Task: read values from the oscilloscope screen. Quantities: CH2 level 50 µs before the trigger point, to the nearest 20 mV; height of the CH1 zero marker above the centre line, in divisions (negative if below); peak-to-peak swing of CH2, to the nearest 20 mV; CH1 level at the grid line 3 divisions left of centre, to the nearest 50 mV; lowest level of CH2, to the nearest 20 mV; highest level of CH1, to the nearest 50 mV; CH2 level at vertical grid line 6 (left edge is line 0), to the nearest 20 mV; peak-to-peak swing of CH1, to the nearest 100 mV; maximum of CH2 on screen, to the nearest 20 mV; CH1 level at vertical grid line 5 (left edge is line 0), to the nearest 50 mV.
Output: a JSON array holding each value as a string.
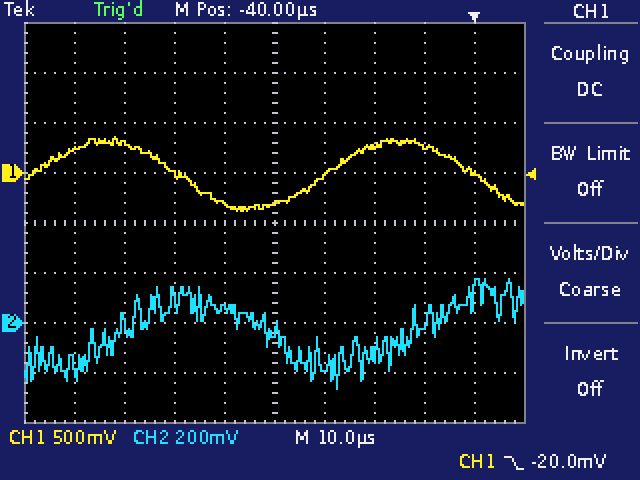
["60 mV", "+1.0 div", "440 mV", "300 mV", "-260 mV", "350 mV", "-180 mV", "700 mV", "180 mV", "-300 mV"]
